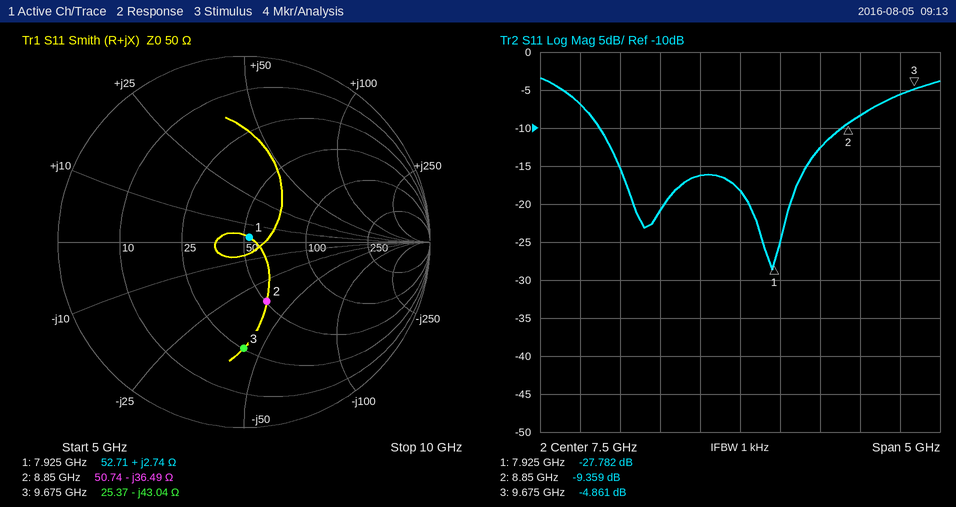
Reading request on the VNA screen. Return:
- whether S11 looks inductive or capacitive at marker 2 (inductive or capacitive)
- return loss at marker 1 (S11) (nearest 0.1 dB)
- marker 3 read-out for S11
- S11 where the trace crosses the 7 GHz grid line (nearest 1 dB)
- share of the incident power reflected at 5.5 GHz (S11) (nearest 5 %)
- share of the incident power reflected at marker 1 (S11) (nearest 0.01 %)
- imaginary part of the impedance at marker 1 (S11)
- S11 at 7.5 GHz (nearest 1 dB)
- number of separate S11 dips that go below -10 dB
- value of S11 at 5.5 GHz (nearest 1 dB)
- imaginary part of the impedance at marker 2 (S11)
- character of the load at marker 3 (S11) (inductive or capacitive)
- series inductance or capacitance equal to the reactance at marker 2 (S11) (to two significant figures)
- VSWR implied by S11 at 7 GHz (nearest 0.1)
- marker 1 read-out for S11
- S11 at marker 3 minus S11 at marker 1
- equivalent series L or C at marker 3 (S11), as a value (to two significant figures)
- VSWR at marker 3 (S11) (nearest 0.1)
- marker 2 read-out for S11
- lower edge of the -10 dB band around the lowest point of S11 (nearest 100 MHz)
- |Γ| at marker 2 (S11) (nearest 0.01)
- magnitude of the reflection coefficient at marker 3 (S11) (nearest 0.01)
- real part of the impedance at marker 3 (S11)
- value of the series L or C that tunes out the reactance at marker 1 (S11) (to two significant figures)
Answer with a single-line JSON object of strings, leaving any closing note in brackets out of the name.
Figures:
{"whether S11 looks inductive or capacitive at marker 2": "capacitive", "return loss at marker 1 (S11)": "28.5 dB", "marker 3 read-out for S11": "-4.861 dB", "S11 where the trace crosses the 7 GHz grid line": "-16 dB", "share of the incident power reflected at 5.5 GHz (S11)": "20 %", "share of the incident power reflected at marker 1 (S11)": "0.17 %", "imaginary part of the impedance at marker 1": "+2.74 Ω", "S11 at 7.5 GHz": "-18 dB", "number of separate S11 dips that go below -10 dB": "2", "value of S11 at 5.5 GHz": "-7 dB", "imaginary part of the impedance at marker 2": "-36.49 Ω", "character of the load at marker 3 (S11)": "capacitive", "series inductance or capacitance equal to the reactance at marker 2 (S11)": "490 fF", "VSWR implied by S11 at 7 GHz": "1.4", "marker 1 read-out for S11": "-27.782 dB", "S11 at marker 3 minus S11 at marker 1": "22.921 dB", "equivalent series L or C at marker 3 (S11), as a value": "380 fF", "VSWR at marker 3 (S11)": "3.7", "marker 2 read-out for S11": "-9.359 dB", "lower edge of the -10 dB band around the lowest point of S11": "5.7 GHz", "|Γ| at marker 2 (S11)": "0.34", "magnitude of the reflection coefficient at marker 3 (S11)": "0.57", "real part of the impedance at marker 3": "25.37 Ω", "value of the series L or C that tunes out the reactance at marker 1 (S11)": "7.3 pF"}
